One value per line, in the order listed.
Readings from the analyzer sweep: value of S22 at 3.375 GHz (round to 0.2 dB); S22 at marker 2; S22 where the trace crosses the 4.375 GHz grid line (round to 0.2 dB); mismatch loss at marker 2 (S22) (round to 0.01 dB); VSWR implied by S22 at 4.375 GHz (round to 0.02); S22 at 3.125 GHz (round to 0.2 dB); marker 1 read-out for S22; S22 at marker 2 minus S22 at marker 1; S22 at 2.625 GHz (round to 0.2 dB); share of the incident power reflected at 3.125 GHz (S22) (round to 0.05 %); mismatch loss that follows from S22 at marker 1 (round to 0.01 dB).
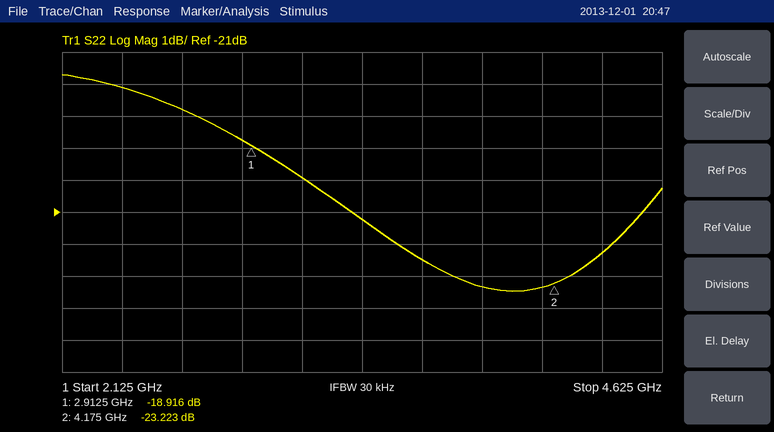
-21.2 dB
-23.223 dB
-22.2 dB
0.02 dB
1.16
-20.0 dB
-18.916 dB
-4.307 dB
-17.8 dB
1.00 %
0.06 dB
